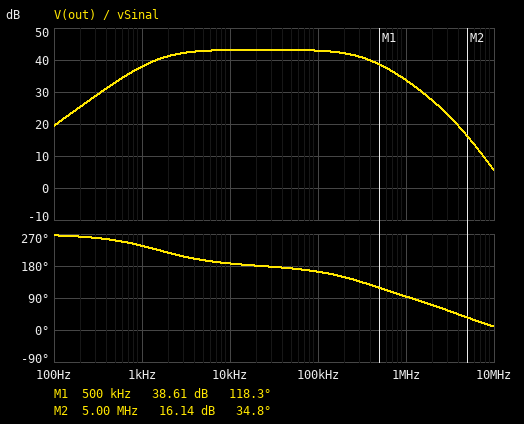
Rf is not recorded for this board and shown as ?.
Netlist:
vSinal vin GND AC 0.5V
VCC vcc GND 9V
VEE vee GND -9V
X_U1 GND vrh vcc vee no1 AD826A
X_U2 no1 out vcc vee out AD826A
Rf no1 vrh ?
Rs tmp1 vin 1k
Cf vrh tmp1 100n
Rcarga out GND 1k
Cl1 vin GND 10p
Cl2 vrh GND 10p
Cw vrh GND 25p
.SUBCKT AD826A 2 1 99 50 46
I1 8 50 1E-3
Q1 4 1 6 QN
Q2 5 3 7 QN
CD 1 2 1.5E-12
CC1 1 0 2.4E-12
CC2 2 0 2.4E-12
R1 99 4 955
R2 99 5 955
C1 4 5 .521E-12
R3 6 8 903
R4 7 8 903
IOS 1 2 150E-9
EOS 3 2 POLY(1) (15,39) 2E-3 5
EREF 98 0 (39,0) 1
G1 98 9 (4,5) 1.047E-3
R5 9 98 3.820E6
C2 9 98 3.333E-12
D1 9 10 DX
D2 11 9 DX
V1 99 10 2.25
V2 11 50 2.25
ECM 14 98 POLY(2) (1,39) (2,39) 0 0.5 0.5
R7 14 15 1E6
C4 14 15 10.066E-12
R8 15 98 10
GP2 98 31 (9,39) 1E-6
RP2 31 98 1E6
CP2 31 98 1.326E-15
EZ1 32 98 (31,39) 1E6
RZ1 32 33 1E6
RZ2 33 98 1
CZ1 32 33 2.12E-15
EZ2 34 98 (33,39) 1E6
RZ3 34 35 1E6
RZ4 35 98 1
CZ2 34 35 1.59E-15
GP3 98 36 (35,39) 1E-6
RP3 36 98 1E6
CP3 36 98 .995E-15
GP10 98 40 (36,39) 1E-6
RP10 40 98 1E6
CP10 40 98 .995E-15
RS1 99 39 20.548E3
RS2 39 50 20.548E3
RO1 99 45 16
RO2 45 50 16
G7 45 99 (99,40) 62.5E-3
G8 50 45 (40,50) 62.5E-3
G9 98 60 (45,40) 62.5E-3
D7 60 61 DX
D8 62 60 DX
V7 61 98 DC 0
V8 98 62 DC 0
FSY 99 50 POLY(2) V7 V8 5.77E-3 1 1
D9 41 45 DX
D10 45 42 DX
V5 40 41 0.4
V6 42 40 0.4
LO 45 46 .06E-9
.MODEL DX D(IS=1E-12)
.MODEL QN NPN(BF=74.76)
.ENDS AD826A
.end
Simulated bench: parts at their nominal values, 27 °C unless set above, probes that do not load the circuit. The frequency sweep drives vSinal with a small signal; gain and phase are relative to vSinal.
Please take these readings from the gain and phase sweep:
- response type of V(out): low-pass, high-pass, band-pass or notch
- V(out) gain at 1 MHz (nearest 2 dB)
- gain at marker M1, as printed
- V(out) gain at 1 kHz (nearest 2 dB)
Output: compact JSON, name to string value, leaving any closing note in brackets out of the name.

{"response type of V(out): low-pass, high-pass, band-pass or notch": "band-pass", "V(out) gain at 1 MHz": "34 dB", "gain at marker M1, as printed": "38.61 dB", "V(out) gain at 1 kHz": "38 dB"}
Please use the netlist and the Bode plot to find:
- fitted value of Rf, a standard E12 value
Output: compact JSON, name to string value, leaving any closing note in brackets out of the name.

{"fitted value of Rf, a standard E12 value": "150 kΩ"}
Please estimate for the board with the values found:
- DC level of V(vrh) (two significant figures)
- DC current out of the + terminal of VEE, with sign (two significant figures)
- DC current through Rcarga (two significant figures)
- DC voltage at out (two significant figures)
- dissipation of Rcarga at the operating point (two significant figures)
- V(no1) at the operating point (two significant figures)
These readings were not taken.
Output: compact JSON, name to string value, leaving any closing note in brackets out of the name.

{"DC level of V(vrh)": "1.7 mV", "DC current out of the + terminal of VEE, with sign": "-14 mA", "DC current through Rcarga": "1.0 mA", "DC voltage at out": "1.0 V", "dissipation of Rcarga at the operating point": "1.0 mW", "V(no1) at the operating point": "1.0 V"}
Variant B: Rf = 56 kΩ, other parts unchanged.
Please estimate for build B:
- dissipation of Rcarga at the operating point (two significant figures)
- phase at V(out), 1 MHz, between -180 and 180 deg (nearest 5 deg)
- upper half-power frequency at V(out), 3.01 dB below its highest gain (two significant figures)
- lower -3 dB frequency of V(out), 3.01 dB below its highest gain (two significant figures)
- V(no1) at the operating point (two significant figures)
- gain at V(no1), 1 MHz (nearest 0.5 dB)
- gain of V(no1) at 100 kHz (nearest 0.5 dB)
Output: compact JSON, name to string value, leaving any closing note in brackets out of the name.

{"dissipation of Rcarga at the operating point": "150 µW", "phase at V(out), 1 MHz, between -180 and 180 deg": "120 deg", "upper half-power frequency at V(out), 3.01 dB below its highest gain": "1.1 MHz", "lower -3 dB frequency of V(out), 3.01 dB below its highest gain": "1.6 kHz", "V(no1) at the operating point": "380 mV", "gain at V(no1), 1 MHz": "32.0 dB", "gain of V(no1) at 100 kHz": "35.0 dB"}
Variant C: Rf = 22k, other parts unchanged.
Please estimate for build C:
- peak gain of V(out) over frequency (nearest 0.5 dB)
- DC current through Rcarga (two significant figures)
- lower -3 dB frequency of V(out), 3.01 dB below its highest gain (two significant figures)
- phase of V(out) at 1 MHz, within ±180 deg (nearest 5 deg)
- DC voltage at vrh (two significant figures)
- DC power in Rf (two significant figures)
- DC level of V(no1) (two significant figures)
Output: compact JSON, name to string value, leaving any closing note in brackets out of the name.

{"peak gain of V(out) over frequency": "27.0 dB", "DC current through Rcarga": "150 µA", "lower -3 dB frequency of V(out), 3.01 dB below its highest gain": "1.6 kHz", "phase of V(out) at 1 MHz, within ±180 deg": "150 deg", "DC voltage at vrh": "2.0 mV", "DC power in Rf": "1.0 µW", "DC level of V(no1)": "150 mV"}
